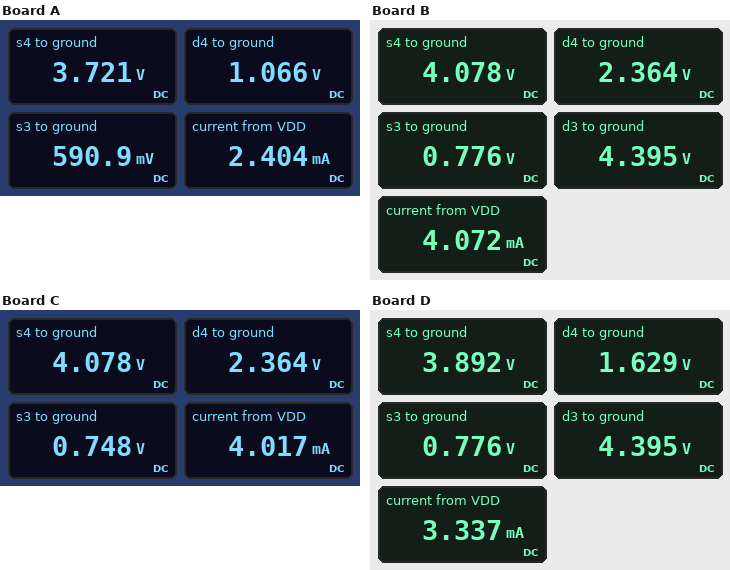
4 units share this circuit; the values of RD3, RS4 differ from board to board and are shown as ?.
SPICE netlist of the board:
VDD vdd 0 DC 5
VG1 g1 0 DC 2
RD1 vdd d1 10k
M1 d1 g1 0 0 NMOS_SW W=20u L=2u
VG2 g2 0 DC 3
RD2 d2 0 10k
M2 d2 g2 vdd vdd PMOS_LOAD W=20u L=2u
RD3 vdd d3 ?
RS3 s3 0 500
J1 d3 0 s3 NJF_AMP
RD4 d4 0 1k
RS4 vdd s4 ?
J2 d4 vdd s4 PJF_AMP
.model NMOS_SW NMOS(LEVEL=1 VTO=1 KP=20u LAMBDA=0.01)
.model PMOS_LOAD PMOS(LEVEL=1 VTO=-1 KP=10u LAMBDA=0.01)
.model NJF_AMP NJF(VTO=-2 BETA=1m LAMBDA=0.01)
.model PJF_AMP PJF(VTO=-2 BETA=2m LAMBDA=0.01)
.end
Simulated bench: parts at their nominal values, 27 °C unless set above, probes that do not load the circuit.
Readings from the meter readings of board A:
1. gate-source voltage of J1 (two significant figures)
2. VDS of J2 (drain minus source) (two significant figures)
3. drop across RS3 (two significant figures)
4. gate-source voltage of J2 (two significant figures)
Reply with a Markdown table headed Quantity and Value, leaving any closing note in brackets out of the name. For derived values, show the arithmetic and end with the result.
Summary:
| Quantity | Value |
|---|---|
| gate-source voltage of J1 | 0 V - 590.9 mV = -590 mV |
| VDS of J2 (drain minus source) | 1.066 V - 3.721 V = -2.7 V |
| drop across RS3 | 590.9 mV = 590 mV |
| gate-source voltage of J2 | 5 V - 3.721 V = 1.3 V |
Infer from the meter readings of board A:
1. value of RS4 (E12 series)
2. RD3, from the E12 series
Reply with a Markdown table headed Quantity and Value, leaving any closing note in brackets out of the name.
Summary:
| Quantity | Value |
|---|---|
| value of RS4 | 1.2 kΩ |
| RD3, from the E12 series | 3.3 kΩ |
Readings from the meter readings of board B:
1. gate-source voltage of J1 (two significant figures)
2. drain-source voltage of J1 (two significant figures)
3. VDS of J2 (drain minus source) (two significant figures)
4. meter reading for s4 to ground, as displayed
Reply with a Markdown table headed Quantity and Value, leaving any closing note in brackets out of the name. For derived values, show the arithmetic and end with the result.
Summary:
| Quantity | Value |
|---|---|
| gate-source voltage of J1 | 0 V - 776 mV = -780 mV |
| drain-source voltage of J1 | 4.395 V - 776 mV = 3.6 V |
| VDS of J2 (drain minus source) | 2.364 V - 4.078 V = -1.7 V |
| meter reading for s4 to ground, as displayed | 4.078 V |
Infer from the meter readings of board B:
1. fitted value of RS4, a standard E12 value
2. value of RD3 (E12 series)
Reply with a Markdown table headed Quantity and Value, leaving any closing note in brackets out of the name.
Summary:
| Quantity | Value |
|---|---|
| fitted value of RS4, a standard E12 value | 390 Ω |
| value of RD3 | 390 Ω |
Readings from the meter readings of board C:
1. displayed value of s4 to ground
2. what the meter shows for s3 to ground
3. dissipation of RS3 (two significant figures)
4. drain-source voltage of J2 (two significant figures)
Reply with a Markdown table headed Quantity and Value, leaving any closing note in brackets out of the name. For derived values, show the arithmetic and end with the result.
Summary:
| Quantity | Value |
|---|---|
| displayed value of s4 to ground | 4.078 V |
| what the meter shows for s3 to ground | 0.748 V |
| dissipation of RS3 | (748 mV)^2 / 500 Ω = 1.1 mW |
| drain-source voltage of J2 | 2.364 V - 4.078 V = -1.7 V |
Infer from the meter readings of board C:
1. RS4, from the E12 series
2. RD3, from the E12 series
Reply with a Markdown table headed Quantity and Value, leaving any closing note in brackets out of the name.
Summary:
| Quantity | Value |
|---|---|
| RS4, from the E12 series | 390 Ω |
| RD3, from the E12 series | 2.2 kΩ |
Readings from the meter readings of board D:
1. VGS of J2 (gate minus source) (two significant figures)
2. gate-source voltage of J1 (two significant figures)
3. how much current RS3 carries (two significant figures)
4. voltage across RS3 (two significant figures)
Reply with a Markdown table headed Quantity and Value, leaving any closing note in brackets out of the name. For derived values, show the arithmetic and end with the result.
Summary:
| Quantity | Value |
|---|---|
| VGS of J2 (gate minus source) | 5 V - 3.892 V = 1.1 V |
| gate-source voltage of J1 | 0 V - 776 mV = -780 mV |
| how much current RS3 carries | (776 mV) / 500 Ω = 1.6 mA |
| voltage across RS3 | 776 mV = 780 mV |
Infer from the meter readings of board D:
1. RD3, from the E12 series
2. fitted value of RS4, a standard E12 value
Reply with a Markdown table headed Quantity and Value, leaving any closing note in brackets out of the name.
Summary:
| Quantity | Value |
|---|---|
| RD3, from the E12 series | 390 Ω |
| fitted value of RS4, a standard E12 value | 680 Ω |
